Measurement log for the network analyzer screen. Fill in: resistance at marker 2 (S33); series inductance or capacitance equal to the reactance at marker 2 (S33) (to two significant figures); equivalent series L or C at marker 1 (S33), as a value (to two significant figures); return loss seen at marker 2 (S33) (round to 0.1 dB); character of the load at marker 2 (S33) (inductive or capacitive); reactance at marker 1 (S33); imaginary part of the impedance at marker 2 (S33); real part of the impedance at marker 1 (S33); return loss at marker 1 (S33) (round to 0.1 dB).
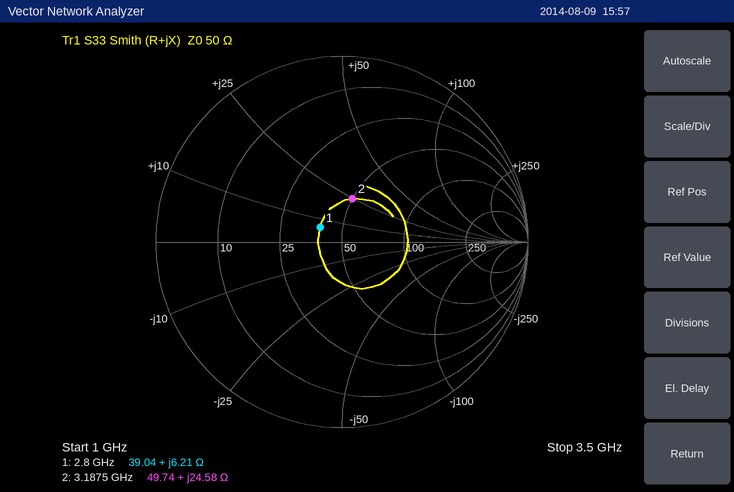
49.74 Ω
1.2 nH
350 pH
12.4 dB
inductive
+6.21 Ω
+24.58 Ω
39.04 Ω
17.0 dB
